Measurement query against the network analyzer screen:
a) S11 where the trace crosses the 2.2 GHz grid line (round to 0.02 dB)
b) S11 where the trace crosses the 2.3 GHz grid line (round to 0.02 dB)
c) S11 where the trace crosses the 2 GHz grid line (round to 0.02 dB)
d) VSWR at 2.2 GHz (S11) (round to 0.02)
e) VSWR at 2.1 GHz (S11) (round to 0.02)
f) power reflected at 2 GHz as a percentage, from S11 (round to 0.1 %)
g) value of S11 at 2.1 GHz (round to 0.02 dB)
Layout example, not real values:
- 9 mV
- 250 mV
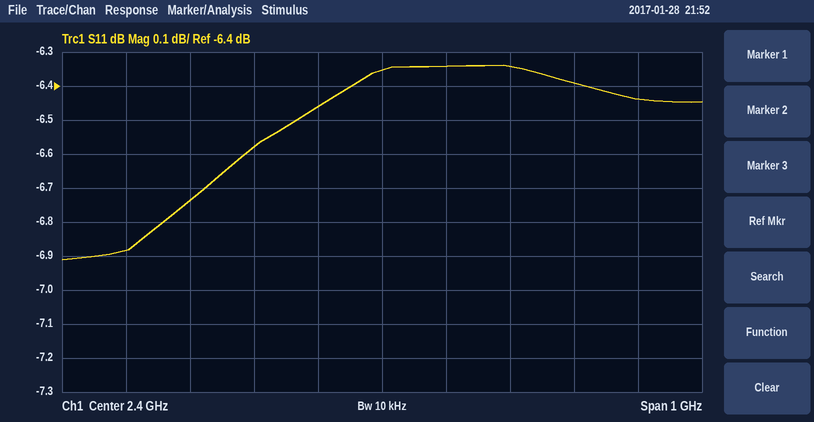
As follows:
- -6.58 dB
- -6.46 dB
- -6.88 dB
- 2.76
- 2.70
- 20.5 %
- -6.74 dB
